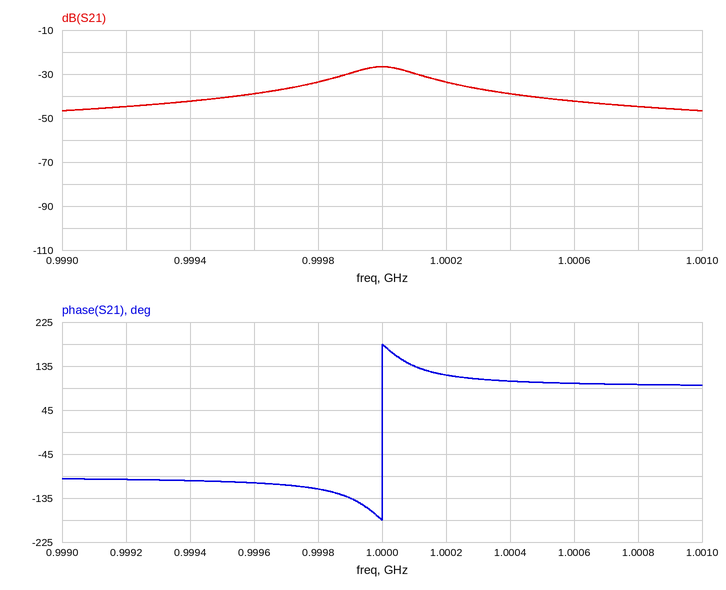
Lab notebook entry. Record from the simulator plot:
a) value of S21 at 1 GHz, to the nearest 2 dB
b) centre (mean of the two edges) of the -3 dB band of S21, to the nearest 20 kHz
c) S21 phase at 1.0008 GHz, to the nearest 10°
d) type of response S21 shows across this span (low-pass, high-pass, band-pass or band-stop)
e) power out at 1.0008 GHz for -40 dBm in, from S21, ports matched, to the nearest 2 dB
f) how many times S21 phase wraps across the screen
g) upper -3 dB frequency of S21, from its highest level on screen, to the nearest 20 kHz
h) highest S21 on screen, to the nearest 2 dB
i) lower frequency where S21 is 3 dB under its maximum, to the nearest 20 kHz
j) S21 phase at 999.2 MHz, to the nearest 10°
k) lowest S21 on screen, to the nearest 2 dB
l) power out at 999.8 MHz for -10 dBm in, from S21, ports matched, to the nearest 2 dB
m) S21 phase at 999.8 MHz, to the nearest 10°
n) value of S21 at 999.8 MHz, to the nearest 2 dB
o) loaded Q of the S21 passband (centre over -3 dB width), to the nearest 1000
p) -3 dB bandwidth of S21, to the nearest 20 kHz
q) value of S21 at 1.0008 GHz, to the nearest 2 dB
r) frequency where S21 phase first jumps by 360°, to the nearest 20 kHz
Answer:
-26 dB
1.00000 GHz
100°
band-pass
-84 dBm
1
1.00010 GHz
-26 dB
999.90 MHz
-100°
-46 dB
-44 dBm
-120°
-34 dB
5000
200 kHz
-44 dB
1.00000 GHz
